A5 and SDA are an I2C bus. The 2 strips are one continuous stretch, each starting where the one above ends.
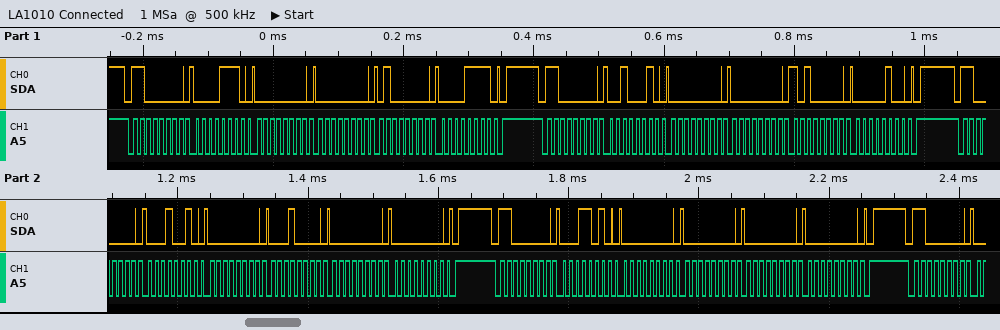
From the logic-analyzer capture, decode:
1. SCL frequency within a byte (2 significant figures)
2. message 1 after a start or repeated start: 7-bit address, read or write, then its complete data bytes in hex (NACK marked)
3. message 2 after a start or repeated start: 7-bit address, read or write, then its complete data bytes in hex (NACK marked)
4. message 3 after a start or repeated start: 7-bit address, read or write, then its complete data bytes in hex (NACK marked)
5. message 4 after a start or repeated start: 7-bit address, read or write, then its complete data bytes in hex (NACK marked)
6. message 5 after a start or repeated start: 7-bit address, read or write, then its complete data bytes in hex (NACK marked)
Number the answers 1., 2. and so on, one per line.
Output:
1. 100 kHz
2. 0x60 write: 0E 00 00 40 0F
3. 0x60 write: 22 00 00 A0 04
4. 0x60 write: 12 00 10 00 00
5. 0x60 write: 1A 00 00 00 00
6. 0x60 write
